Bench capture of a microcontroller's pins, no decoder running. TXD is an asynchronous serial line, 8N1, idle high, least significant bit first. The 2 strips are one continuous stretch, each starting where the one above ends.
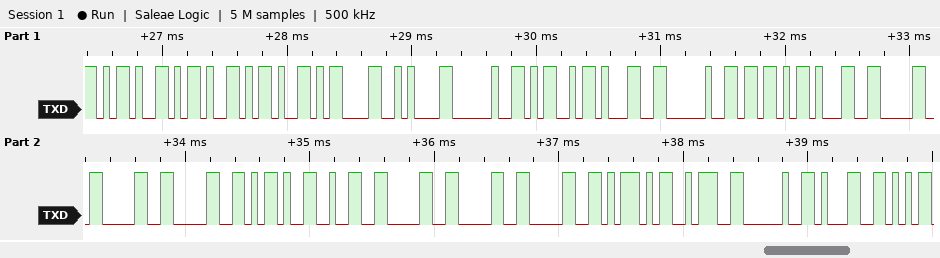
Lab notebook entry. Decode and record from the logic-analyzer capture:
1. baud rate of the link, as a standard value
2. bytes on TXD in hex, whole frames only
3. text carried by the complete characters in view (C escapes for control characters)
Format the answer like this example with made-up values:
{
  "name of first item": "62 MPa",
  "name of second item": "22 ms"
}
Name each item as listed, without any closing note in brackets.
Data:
{
  "baud rate of the link, as a standard value": "19200 baud",
  "bytes on TXD in hex, whole frames only": "2D 2D 2D 0D 0A 20 4D 31 20 5B 31 30 30 30 2D 32 30 30 30 5D 3A 20 31",
  "text carried by the complete characters in view": "\"---\\r\\n M1 [1000-2000]: 1\""
}
